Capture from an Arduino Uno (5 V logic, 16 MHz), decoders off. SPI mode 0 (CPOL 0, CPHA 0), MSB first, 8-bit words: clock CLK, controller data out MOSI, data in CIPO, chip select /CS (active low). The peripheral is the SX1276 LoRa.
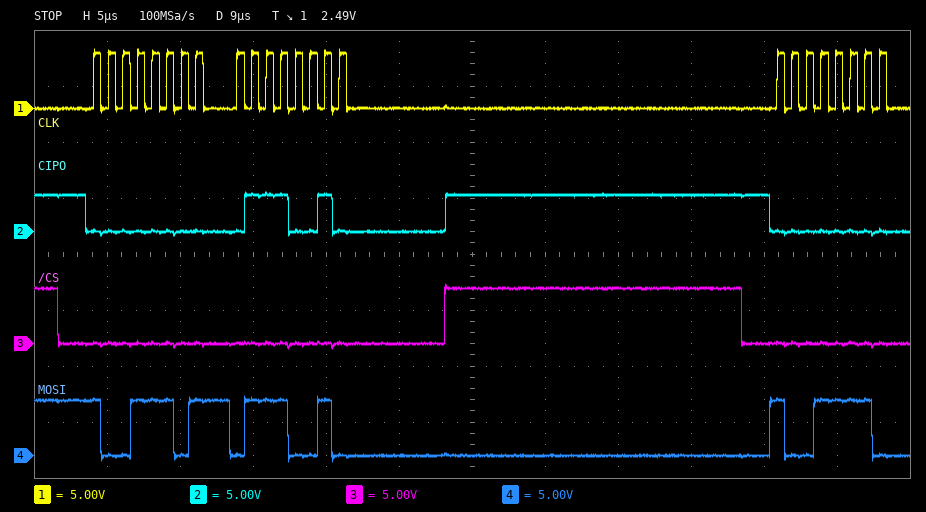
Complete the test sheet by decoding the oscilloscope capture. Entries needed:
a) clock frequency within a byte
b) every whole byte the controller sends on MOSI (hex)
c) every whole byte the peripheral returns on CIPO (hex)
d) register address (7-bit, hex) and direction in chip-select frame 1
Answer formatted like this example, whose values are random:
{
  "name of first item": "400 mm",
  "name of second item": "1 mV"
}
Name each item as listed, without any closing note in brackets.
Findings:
{
  "clock frequency within a byte": "1 MHz",
  "every whole byte the controller sends on MOSI": "9D 72 9E",
  "every whole byte the peripheral returns on CIPO": "00 72 00",
  "register address (7-bit, hex) and direction in chip-select frame 1": "0x1D write"
}
